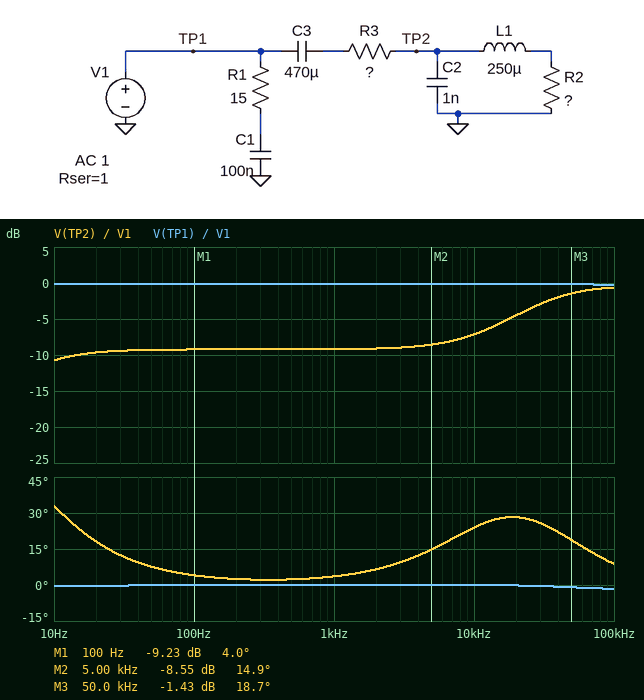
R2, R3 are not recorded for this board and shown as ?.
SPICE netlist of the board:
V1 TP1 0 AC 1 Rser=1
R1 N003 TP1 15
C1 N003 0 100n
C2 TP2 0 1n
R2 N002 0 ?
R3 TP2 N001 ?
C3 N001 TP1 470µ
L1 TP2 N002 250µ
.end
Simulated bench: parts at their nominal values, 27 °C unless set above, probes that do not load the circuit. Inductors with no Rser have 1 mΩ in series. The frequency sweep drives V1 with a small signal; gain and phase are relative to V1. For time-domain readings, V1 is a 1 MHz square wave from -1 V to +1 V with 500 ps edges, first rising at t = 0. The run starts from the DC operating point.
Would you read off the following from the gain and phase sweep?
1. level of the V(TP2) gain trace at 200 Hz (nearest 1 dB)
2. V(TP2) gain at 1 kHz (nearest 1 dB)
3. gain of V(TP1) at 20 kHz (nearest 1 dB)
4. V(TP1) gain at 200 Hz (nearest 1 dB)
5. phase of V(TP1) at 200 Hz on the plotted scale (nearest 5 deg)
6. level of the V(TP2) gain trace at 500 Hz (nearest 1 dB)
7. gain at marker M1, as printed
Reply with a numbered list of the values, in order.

1. -9 dB
2. -9 dB
3. 0 dB
4. 0 dB
5. 0 deg
6. -9 dB
7. -9.23 dB
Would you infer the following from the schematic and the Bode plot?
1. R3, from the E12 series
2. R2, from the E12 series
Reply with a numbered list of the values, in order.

1. 33 Ω
2. 18 Ω
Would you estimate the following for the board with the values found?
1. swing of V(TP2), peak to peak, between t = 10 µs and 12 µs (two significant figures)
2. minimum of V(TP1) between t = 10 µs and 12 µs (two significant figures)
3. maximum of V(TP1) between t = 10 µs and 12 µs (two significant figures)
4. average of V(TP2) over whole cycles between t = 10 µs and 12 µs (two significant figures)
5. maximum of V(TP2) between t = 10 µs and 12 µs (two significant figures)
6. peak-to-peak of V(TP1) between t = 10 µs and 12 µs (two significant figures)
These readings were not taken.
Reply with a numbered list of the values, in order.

1. 1.9 V
2. -960 mV
3. 930 mV
4. 420 mV
5. 1.4 V
6. 1.9 V
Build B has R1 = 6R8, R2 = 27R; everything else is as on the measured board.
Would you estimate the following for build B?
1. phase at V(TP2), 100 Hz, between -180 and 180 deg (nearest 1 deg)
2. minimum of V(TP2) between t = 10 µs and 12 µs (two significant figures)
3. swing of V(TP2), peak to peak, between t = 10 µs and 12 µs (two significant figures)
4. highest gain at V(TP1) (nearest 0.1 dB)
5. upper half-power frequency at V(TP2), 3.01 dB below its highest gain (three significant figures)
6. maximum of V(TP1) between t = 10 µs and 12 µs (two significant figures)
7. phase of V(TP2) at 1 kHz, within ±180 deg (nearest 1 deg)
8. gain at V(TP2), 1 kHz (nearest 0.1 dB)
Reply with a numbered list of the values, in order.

1. 3 deg
2. -410 mV
3. 1.8 V
4. 0 dB
5. 4.05 MHz
6. 900 mV
7. 2 deg
8. -7.1 dB
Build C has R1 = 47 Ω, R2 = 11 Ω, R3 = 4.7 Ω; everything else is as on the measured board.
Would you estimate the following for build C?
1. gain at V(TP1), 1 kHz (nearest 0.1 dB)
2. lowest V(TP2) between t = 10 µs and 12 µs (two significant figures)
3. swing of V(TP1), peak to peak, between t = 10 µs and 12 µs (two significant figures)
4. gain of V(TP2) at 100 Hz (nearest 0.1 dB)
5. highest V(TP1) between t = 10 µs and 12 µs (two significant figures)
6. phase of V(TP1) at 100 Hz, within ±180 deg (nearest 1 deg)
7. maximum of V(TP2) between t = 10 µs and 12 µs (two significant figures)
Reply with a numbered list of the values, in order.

1. -0.5 dB
2. -170 mV
3. 2.0 V
4. -3.8 dB
5. 950 mV
6. -1 deg
7. 1.8 V
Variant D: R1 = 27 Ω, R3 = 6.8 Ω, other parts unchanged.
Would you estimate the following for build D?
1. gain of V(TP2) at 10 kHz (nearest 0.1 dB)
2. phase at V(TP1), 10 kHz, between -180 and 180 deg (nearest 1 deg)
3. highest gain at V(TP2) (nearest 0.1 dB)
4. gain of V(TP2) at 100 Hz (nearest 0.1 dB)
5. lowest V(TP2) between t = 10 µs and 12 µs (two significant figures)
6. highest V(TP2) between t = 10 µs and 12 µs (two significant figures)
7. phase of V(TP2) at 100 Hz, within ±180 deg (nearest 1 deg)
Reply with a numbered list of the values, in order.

1. -2.0 dB
2. 1 deg
3. -0.3 dB
4. -3.2 dB
5. -180 mV
6. 1.8 V
7. 8 deg
